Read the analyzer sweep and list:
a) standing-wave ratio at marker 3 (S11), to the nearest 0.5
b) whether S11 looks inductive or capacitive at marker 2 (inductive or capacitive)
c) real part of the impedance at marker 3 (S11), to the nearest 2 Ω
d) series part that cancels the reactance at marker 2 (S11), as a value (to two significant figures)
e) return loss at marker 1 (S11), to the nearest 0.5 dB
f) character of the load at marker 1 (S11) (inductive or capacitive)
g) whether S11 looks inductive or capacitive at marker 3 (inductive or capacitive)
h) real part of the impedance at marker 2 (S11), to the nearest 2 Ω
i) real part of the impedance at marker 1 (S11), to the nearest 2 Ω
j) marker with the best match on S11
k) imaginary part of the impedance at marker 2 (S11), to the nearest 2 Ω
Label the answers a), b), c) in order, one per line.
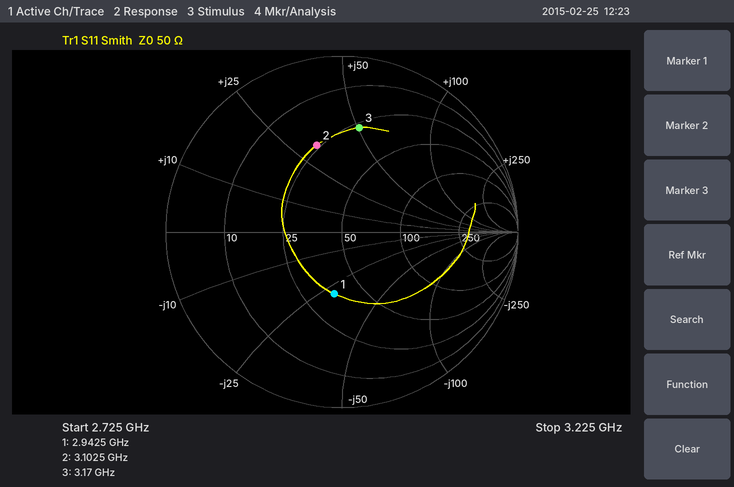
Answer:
a) 4.0
b) inductive
c) 28 Ω
d) 1.6 pF
e) 9.0 dB
f) capacitive
g) inductive
h) 24 Ω
i) 36 Ω
j) marker 1
k) +32 Ω
